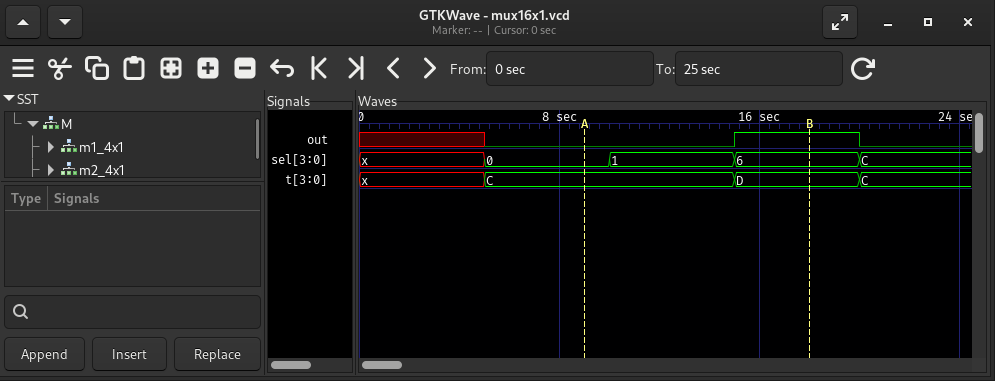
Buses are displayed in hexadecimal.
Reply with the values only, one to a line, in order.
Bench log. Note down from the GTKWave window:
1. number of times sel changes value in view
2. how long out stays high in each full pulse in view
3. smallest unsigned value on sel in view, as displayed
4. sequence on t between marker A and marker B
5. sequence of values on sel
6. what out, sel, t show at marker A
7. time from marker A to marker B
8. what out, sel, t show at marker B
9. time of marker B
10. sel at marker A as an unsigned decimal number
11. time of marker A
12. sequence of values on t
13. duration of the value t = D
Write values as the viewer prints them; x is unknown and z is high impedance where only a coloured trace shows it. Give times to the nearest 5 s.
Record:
4
5 s
0
C, D
x, 0, 1, 6, C
out=0, sel=0, t=C
10 s
out=1, sel=6, t=D
20 s
0
10 s
x, C, D, C
5 s
